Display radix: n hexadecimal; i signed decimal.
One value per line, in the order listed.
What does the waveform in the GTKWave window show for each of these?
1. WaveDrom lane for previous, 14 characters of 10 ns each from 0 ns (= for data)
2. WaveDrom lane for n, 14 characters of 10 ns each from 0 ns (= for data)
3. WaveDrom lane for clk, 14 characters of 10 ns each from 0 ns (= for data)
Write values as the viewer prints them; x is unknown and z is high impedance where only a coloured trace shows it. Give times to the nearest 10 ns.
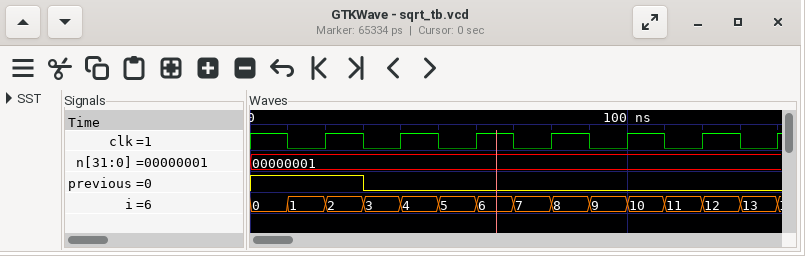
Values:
{name: 'previous', wave: '1..0..........'}
{name: 'n', wave: '=.............', data: '00000001'}
{name: 'clk', wave: '10101010101010'}
